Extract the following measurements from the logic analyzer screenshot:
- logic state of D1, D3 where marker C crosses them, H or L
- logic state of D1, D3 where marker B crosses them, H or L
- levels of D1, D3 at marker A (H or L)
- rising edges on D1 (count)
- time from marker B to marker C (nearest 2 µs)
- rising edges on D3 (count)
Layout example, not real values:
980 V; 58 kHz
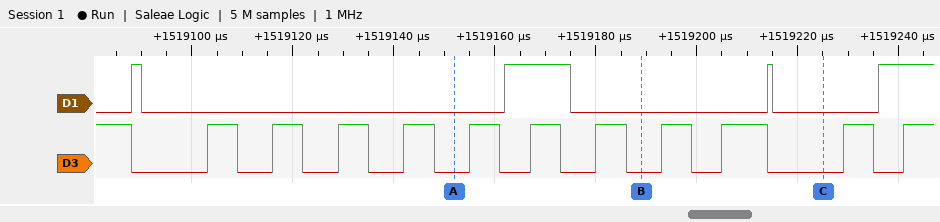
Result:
D1=L, D3=L; D1=L, D3=L; D1=L, D3=L; 4; 36 µs; 11
